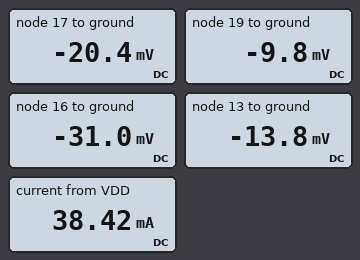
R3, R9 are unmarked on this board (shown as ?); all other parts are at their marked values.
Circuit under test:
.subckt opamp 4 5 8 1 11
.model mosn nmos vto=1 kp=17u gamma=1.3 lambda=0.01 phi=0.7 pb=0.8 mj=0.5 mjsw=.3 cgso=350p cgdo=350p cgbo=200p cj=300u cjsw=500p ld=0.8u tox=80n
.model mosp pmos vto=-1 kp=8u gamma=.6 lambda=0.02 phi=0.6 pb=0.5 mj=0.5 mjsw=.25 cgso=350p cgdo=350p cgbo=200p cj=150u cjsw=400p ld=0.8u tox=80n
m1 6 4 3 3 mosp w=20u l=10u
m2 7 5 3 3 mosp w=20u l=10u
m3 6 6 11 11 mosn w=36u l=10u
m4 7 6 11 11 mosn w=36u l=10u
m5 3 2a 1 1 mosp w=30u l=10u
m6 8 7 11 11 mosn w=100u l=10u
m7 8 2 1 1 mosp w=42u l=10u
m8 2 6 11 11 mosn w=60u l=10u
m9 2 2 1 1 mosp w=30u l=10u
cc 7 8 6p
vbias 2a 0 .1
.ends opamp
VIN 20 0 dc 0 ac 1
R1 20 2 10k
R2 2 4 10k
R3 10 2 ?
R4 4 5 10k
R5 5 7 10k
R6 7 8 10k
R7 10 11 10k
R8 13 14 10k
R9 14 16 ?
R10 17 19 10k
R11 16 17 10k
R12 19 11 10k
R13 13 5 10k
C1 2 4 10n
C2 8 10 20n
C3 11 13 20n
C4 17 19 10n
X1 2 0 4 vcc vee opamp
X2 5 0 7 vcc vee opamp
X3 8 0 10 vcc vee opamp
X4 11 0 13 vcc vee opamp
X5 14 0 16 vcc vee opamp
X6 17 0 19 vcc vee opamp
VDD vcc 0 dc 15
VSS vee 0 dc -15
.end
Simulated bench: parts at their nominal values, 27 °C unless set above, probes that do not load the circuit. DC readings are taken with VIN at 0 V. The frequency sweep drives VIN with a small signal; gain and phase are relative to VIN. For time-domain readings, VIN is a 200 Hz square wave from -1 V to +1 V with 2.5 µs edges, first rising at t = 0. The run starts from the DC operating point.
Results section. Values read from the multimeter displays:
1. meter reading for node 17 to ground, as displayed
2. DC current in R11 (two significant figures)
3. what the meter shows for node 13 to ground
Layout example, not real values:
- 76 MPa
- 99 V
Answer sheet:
- -20.4 mV
- 1.1 µA
- -13.8 mV
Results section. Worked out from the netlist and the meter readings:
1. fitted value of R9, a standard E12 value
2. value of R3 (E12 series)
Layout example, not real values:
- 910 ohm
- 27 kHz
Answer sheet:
- 18 kΩ
- 8.2 kΩ
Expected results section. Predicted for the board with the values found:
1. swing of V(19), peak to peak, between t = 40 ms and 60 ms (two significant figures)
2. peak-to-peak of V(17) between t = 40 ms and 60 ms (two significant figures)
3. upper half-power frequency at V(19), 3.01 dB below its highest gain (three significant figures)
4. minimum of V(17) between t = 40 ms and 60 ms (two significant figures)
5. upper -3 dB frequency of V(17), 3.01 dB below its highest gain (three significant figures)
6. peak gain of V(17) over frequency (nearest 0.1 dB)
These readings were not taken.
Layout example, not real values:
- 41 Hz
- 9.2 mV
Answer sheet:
- 1.3 V
- 32 mV
- 1.57 kHz
- -37 mV
- 1.61 kHz
- -37.7 dB
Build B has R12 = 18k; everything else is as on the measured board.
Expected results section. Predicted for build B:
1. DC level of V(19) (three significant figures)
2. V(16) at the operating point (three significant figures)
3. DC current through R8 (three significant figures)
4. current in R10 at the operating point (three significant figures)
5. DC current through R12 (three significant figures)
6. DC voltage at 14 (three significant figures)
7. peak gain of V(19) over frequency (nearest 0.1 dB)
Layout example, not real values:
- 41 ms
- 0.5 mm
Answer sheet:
- -5.57 mV
- -35.3 mV
- 859 nA
- 1.49 µA
- 821 nA
- -19.8 mV
- -2.8 dB
